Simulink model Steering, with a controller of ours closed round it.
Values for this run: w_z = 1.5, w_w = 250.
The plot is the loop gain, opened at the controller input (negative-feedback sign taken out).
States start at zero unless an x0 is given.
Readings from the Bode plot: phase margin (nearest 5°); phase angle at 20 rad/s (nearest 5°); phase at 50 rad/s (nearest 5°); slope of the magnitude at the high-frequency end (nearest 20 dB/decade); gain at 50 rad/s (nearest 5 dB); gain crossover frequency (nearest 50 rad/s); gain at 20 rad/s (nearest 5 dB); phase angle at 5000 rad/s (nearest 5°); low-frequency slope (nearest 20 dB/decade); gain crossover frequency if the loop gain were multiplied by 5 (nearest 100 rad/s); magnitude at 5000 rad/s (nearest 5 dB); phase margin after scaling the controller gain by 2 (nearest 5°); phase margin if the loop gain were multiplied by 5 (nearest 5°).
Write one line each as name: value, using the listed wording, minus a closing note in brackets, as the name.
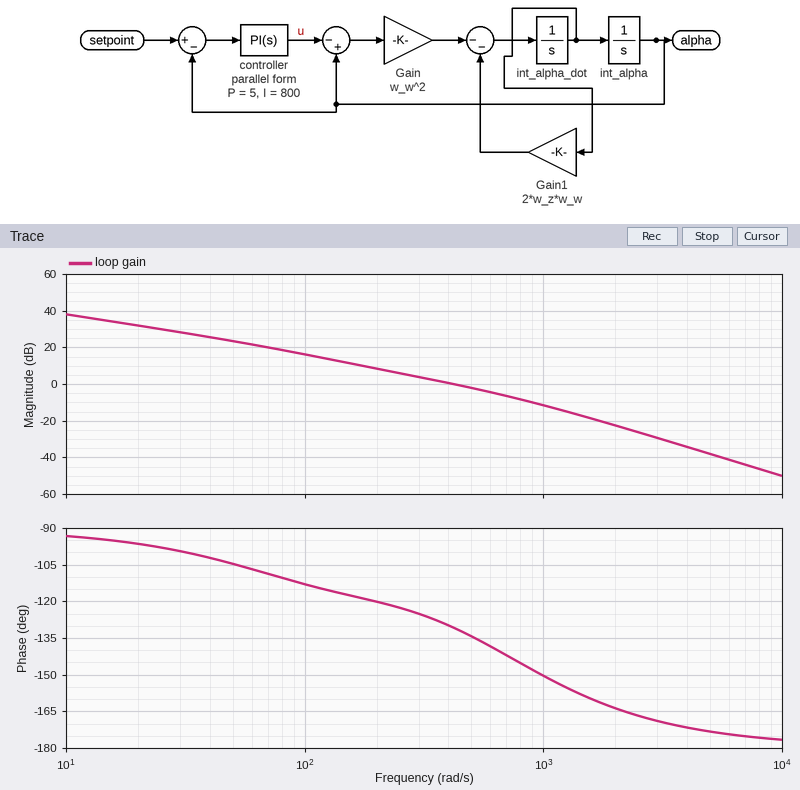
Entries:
phase margin: 50°
phase angle at 20 rad/s: -95°
phase at 50 rad/s: -105°
slope of the magnitude at the high-frequency end: -40 dB/decade
gain at 50 rad/s: 25 dB
gain crossover frequency: 400 rad/s
gain at 20 rad/s: 30 dB
phase angle at 5000 rad/s: -175°
low-frequency slope: -20 dB/decade
gain crossover frequency if the loop gain were multiplied by 5: 1200 rad/s
magnitude at 5000 rad/s: -40 dB
phase margin after scaling the controller gain by 2: 40°
phase margin if the loop gain were multiplied by 5: 25°
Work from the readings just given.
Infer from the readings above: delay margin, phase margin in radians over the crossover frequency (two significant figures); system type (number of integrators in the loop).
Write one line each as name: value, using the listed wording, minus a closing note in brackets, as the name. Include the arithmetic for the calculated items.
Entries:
delay margin, phase margin in radians over the crossover frequency: 50 × π / 180 / 400 = 0.0022 s
system type: 1
